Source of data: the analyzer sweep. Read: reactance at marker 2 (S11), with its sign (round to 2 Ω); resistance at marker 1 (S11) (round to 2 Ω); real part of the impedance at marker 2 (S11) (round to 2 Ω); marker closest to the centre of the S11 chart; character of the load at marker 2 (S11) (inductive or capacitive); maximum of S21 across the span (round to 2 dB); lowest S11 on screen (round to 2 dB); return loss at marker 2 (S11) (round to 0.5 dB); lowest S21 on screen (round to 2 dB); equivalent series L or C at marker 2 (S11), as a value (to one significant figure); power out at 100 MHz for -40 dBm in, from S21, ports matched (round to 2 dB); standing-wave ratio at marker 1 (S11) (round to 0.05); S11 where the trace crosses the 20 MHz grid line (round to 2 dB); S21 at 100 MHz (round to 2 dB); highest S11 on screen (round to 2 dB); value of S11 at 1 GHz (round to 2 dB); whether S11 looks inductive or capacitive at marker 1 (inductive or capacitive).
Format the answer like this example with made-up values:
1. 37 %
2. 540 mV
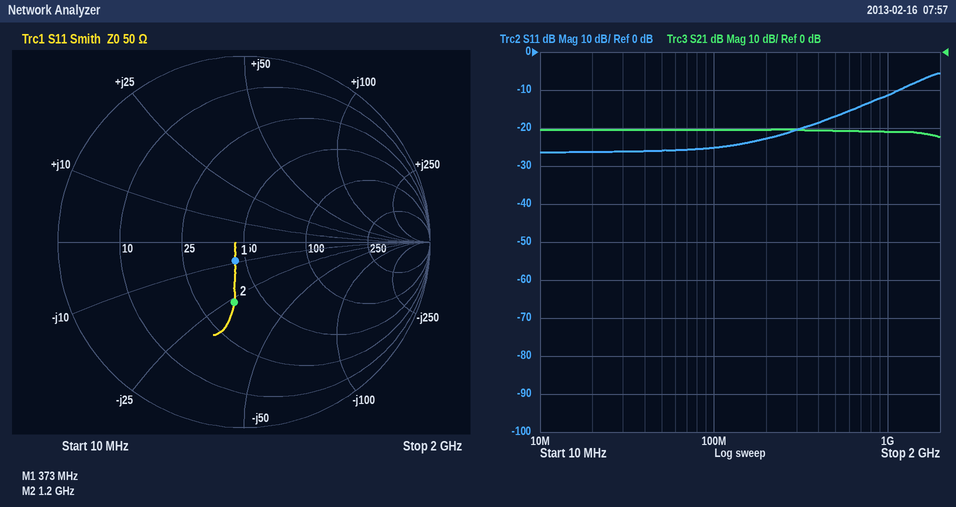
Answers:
1. -26 Ω
2. 44 Ω
3. 36 Ω
4. marker 1
5. capacitive
6. -20 dB
7. -26 dB
8. 9.5 dB
9. -22 dB
10. 5 pF
11. -60 dBm
12. 1.25
13. -26 dB
14. -20 dB
15. -6 dB
16. -12 dB
17. capacitive
